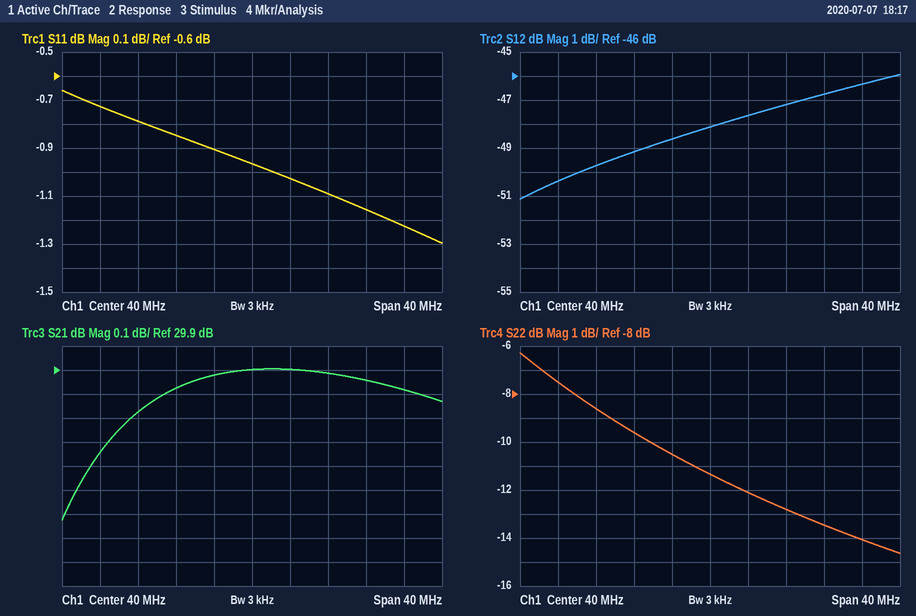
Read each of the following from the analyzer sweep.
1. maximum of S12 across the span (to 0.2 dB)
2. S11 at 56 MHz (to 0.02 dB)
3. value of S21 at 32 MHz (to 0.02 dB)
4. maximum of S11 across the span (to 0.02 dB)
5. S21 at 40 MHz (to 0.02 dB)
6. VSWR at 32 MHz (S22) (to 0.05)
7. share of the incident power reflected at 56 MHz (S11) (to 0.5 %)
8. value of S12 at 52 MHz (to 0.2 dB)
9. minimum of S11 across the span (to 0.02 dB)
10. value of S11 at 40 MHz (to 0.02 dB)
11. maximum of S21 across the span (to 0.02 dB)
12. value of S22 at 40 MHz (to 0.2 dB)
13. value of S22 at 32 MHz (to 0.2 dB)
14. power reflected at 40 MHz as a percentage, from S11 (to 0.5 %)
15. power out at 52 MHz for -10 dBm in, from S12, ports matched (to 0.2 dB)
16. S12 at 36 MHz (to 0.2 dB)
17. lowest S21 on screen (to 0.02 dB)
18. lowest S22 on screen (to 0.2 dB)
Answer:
-46.0 dB
-1.22 dB
29.82 dB
-0.66 dB
29.90 dB
2.00
75.5 %
-46.8 dB
-1.30 dB
-0.96 dB
29.90 dB
-11.4 dB
-9.6 dB
80.0 %
-56.8 dBm
-48.6 dB
29.28 dB
-14.6 dB
